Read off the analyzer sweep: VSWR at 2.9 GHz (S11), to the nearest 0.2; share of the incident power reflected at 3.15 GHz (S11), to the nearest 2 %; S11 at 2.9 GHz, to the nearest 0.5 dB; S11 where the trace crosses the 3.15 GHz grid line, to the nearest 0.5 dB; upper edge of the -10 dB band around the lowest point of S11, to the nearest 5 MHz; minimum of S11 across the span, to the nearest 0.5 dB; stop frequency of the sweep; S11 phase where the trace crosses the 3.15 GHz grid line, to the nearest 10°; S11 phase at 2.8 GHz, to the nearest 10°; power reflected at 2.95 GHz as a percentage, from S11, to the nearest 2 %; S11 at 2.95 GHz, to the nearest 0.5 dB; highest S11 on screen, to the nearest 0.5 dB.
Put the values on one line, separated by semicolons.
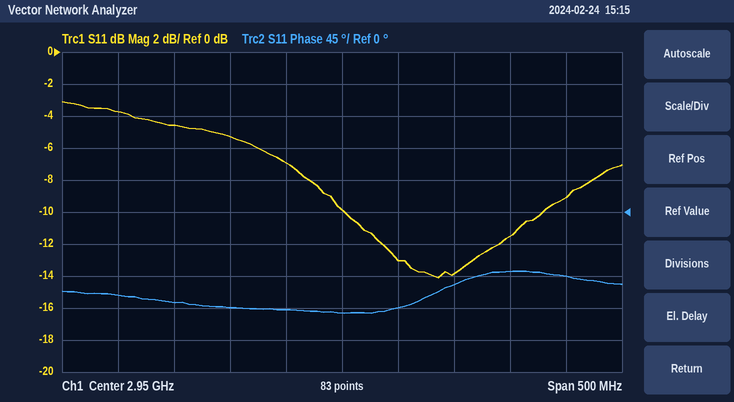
2.6; 12 %; -7.0 dB; -9.0 dB; 3.130 GHz; -14.0 dB; 3.2 GHz; -90°; -130°; 10 %; -10.0 dB; -3.0 dB
